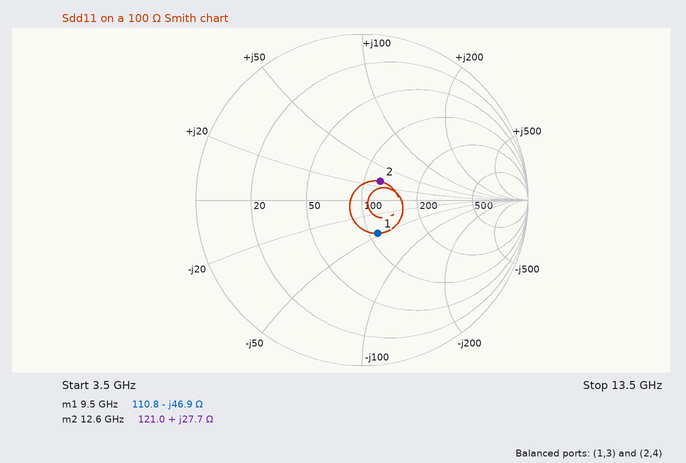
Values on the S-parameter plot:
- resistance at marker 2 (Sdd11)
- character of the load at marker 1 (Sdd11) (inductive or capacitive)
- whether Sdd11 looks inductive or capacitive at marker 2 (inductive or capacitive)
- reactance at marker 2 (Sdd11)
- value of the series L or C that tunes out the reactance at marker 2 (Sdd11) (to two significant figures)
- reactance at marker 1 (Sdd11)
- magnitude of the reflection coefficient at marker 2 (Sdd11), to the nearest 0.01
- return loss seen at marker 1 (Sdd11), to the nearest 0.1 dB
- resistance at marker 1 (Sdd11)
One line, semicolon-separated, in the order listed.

121.0 Ω; capacitive; inductive; +27.7 Ω; 460 fF; -46.9 Ω; 0.16; 13.0 dB; 110.8 Ω
